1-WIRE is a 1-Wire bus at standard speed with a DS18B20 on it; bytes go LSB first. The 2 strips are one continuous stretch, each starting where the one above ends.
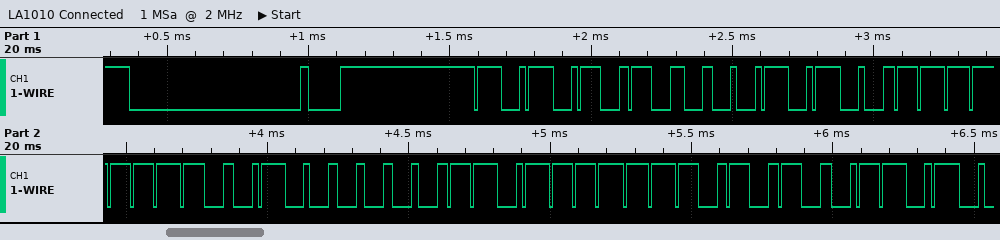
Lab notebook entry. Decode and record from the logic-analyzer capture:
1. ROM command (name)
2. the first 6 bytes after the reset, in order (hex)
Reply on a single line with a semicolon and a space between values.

Match ROM; 55 28 FF 04 F6 57
